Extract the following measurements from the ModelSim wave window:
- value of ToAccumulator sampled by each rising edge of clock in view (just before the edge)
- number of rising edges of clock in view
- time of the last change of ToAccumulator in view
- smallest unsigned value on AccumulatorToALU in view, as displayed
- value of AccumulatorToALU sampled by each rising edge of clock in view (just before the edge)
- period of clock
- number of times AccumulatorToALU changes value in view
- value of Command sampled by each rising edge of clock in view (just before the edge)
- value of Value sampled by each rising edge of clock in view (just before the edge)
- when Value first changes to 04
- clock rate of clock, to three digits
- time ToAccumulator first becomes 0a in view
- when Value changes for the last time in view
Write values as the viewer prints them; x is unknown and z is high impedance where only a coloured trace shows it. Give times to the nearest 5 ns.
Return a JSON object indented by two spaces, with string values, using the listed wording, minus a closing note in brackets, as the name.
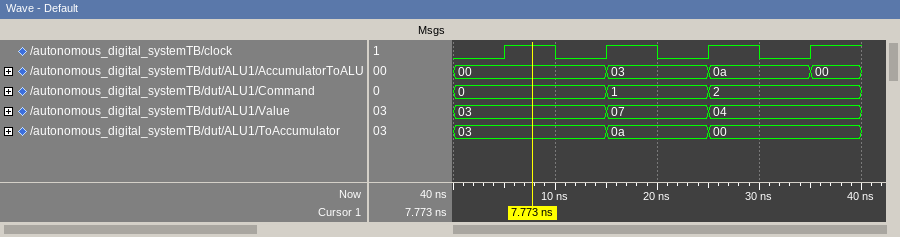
{
  "value of ToAccumulator sampled by each rising edge of clock in view": "03, 03, 0a, 00",
  "number of rising edges of clock in view": "4",
  "time of the last change of ToAccumulator in view": "25 ns",
  "smallest unsigned value on AccumulatorToALU in view, as displayed": "00",
  "value of AccumulatorToALU sampled by each rising edge of clock in view": "00, 00, 03, 0a",
  "period of clock": "10 ns",
  "number of times AccumulatorToALU changes value in view": "3",
  "value of Command sampled by each rising edge of clock in view": "0, 0, 1, 2",
  "value of Value sampled by each rising edge of clock in view": "03, 03, 07, 04",
  "when Value first changes to 04": "25 ns",
  "clock rate of clock, to three digits": "100 MHz",
  "time ToAccumulator first becomes 0a in view": "15 ns",
  "when Value changes for the last time in view": "25 ns"
}
